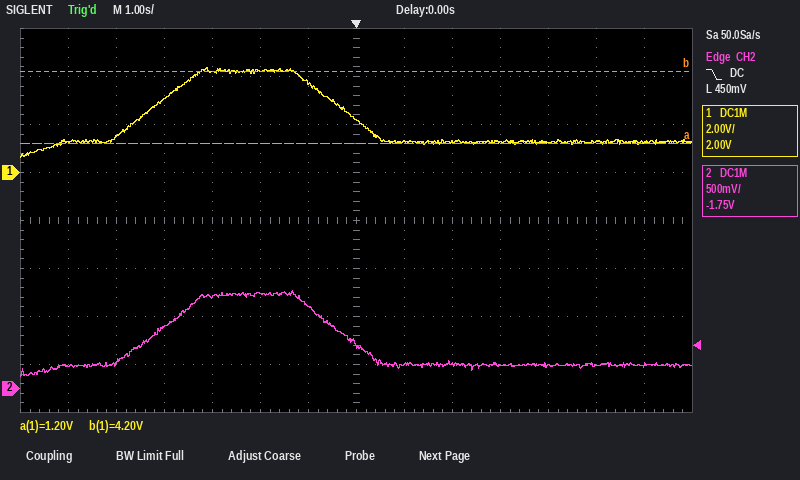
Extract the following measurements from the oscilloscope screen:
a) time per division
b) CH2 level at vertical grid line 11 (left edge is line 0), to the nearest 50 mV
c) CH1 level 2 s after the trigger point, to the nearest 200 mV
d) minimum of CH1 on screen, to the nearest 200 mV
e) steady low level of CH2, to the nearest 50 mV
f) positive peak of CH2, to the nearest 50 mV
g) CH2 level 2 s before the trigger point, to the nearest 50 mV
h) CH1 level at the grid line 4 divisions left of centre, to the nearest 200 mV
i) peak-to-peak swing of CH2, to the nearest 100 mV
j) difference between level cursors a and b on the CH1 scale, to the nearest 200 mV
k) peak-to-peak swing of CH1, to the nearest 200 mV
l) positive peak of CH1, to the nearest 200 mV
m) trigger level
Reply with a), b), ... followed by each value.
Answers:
a) 1 s
b) 250 mV
c) 1.2 V
d) 600 mV
e) 250 mV
f) 1.00 V
g) 1.00 V
h) 3.0 V
i) 900 mV
j) 3.0 V
k) 3.8 V
l) 4.4 V
m) 450 mV
